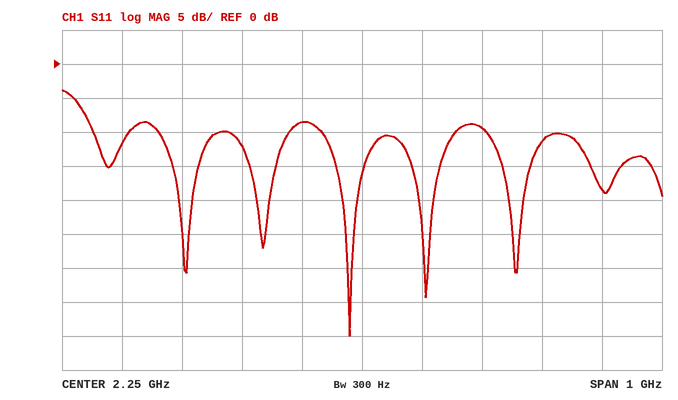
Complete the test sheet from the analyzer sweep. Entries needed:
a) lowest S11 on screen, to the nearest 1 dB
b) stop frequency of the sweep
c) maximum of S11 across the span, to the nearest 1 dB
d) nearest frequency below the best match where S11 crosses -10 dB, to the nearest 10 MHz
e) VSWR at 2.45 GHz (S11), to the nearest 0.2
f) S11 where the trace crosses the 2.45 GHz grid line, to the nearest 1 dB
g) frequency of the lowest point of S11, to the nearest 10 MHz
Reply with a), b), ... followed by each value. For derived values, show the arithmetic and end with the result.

a) -40 dB
b) 2.75 GHz
c) -4 dB
d) 2.18 GHz
e) |Γ| = 10^(-9/20) = 0.3548; VSWR = (1 + 0.3548)/(1 − 0.3548) ≈ 2.10, so 2.0 to the nearest 0.2
f) -9 dB
g) 2.23 GHz
